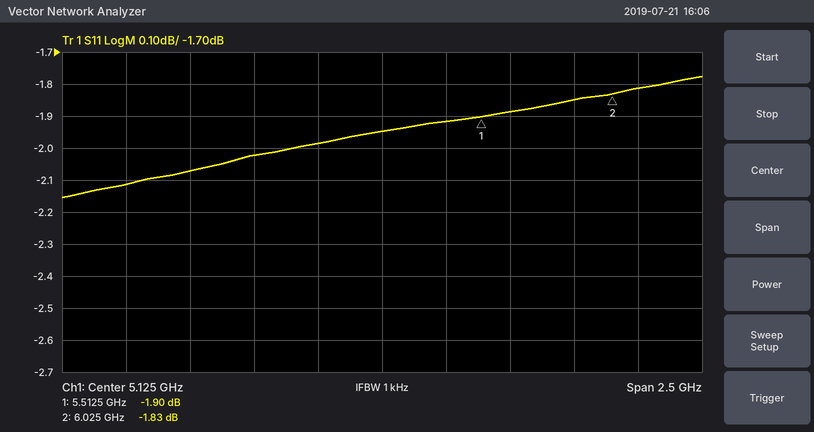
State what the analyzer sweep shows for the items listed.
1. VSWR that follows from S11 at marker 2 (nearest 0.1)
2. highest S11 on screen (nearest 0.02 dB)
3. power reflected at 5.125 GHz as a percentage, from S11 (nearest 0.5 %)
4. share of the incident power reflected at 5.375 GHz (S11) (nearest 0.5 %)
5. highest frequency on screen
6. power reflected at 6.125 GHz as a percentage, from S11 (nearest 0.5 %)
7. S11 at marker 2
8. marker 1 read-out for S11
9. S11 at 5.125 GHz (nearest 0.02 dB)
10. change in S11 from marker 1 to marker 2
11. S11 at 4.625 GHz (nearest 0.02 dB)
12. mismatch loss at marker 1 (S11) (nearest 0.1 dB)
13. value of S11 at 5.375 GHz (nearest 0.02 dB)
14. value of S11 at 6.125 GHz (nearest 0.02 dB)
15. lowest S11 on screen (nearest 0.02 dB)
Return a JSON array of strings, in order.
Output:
["9.5", "-1.78 dB", "64.0 %", "64.5 %", "6.375 GHz", "66.0 %", "-1.83 dB", "-1.90 dB", "-1.94 dB", "0.07 dB", "-2.02 dB", "4.5 dB", "-1.92 dB", "-1.82 dB", "-2.16 dB"]
